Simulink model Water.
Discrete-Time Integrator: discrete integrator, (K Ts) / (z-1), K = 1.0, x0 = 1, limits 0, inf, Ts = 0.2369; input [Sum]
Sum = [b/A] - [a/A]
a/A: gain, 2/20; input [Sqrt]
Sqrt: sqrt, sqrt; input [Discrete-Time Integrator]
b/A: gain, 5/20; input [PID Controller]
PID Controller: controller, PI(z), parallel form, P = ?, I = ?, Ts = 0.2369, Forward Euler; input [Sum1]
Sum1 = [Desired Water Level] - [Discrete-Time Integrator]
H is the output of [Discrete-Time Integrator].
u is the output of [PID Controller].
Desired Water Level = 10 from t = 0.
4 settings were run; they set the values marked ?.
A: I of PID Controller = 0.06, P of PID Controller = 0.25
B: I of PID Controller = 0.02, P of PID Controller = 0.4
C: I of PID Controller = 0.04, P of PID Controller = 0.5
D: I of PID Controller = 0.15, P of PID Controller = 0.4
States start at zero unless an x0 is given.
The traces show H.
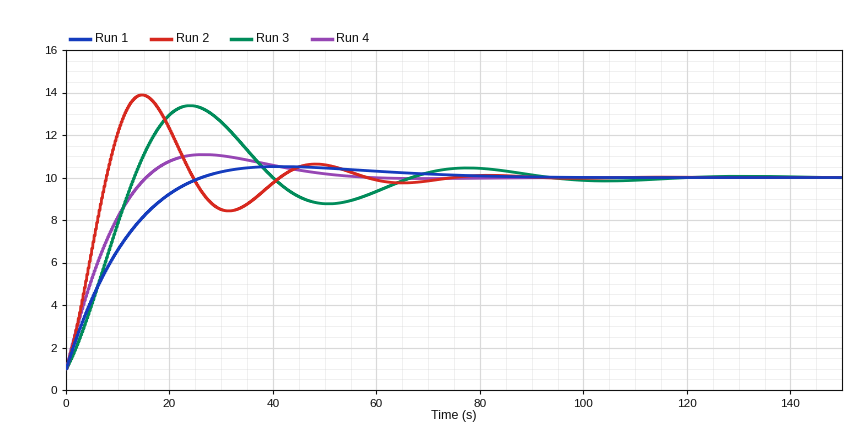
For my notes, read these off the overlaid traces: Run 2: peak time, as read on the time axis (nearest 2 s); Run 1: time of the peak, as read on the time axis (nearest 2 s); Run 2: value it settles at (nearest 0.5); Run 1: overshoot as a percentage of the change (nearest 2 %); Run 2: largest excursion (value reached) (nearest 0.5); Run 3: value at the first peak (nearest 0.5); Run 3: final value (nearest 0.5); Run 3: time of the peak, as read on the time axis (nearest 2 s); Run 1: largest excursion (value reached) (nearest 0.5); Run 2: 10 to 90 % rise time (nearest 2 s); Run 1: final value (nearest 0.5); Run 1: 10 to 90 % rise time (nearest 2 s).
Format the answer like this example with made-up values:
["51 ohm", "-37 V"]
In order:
["14 s", "42 s", "10.0", "6 %", "14.0", "13.5", "10.0", "24 s", "10.5", "6 s", "10.0", "18 s"]
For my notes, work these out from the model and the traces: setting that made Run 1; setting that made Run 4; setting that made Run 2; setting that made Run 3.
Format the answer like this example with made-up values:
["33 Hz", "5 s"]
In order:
["B", "C", "D", "A"]
